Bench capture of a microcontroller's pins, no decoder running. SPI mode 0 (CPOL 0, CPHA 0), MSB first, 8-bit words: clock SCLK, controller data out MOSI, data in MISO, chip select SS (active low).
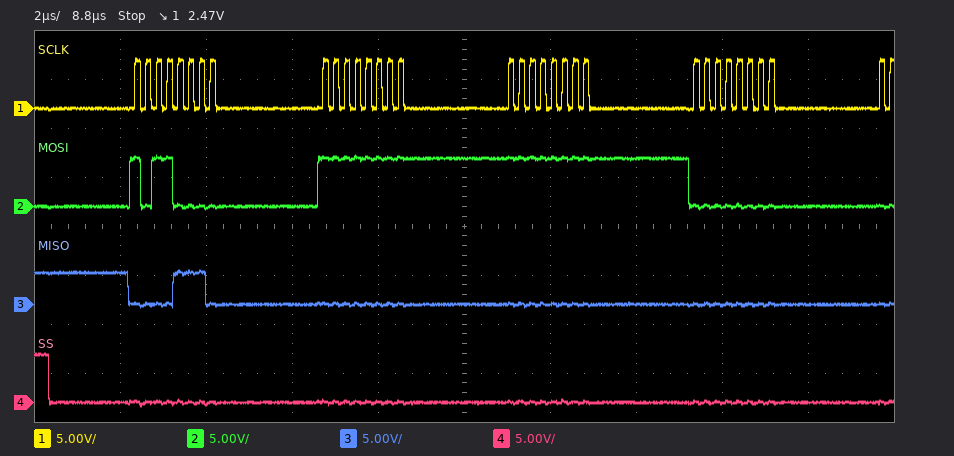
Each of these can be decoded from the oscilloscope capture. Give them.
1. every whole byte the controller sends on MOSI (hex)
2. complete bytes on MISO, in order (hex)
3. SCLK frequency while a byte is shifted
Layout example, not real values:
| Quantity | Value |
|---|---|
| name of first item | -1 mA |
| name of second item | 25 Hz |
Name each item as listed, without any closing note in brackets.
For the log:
| Quantity | Value |
|---|---|
| every whole byte the controller sends on MOSI | B0 FF FF 00 |
| complete bytes on MISO, in order | 0E 00 00 00 |
| SCLK frequency while a byte is shifted | 4 MHz |
